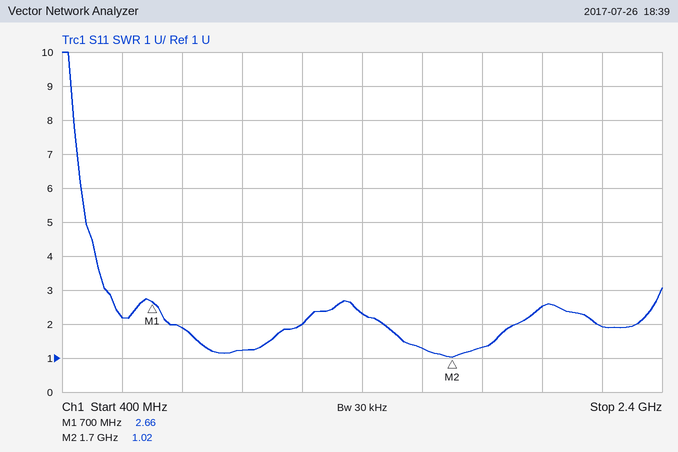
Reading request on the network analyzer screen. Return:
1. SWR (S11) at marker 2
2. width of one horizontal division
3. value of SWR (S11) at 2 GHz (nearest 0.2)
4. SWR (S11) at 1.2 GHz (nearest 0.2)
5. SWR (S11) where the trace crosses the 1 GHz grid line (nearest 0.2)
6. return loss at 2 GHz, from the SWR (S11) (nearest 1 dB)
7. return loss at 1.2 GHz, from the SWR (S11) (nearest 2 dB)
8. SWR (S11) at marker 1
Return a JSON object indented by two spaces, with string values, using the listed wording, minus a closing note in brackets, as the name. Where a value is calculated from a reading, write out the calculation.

{
  "SWR (S11) at marker 2": "1.02",
  "width of one horizontal division": "200 MHz",
  "value of SWR (S11) at 2 GHz": "2.6",
  "SWR (S11) at 1.2 GHz": "2.0",
  "SWR (S11) where the trace crosses the 1 GHz grid line": "1.2",
  "return loss at 2 GHz, from the SWR (S11)": "−20 log10((2.6 − 1)/(2.6 + 1)) ≈ 7 dB",
  "return loss at 1.2 GHz, from the SWR (S11)": "−20 log10((2 − 1)/(2 + 1)) ≈ 10 dB",
  "SWR (S11) at marker 1": "2.66"
}
